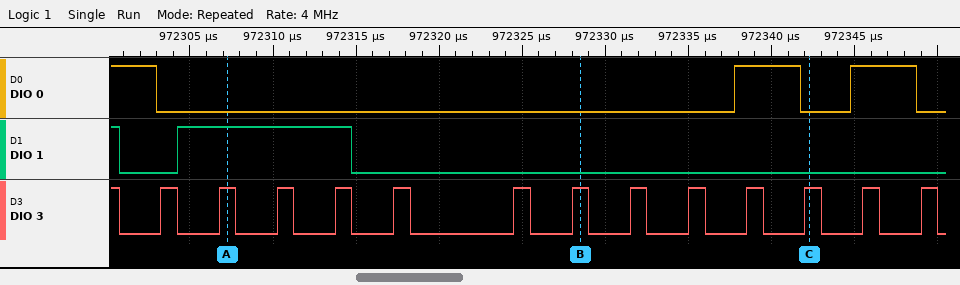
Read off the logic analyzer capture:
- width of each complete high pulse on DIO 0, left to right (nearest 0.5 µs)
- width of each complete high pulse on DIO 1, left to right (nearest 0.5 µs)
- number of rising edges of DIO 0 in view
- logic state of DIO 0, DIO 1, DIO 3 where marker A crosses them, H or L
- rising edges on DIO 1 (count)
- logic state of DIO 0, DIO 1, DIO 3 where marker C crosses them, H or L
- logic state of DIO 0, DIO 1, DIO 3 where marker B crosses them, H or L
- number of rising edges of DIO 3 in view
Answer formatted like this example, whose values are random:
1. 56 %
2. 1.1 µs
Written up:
1. 4 µs, 4 µs
2. 10.5 µs
3. 2
4. DIO 0=L, DIO 1=H, DIO 3=H
5. 1
6. DIO 0=L, DIO 1=L, DIO 3=H
7. DIO 0=L, DIO 1=L, DIO 3=H
8. 13
